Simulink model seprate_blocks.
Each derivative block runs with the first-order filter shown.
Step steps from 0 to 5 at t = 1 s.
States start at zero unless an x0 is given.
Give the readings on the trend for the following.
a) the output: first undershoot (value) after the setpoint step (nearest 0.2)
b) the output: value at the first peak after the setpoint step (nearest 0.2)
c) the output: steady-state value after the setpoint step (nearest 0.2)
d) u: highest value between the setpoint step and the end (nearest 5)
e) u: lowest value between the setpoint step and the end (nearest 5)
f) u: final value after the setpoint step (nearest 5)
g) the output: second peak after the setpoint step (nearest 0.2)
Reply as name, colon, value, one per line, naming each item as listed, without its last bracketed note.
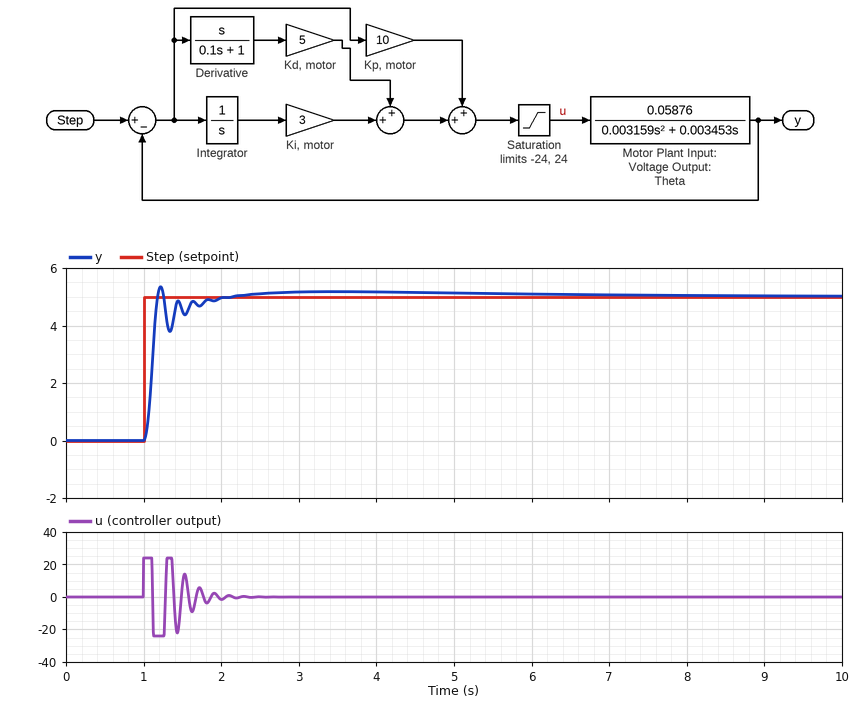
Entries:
the output: first undershoot (value) after the setpoint step: 3.8
the output: value at the first peak after the setpoint step: 5.4
the output: steady-state value after the setpoint step: 5.0
u: highest value between the setpoint step and the end: 25
u: lowest value between the setpoint step and the end: -25
u: final value after the setpoint step: 0
the output: second peak after the setpoint step: 4.8
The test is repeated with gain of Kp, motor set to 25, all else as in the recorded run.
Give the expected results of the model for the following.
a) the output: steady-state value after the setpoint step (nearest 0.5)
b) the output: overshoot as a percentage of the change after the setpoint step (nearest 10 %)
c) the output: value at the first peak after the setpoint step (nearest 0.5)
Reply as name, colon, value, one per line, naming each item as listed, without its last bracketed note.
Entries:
the output: steady-state value after the setpoint step: 5.0
the output: overshoot as a percentage of the change after the setpoint step: 20 %
the output: value at the first peak after the setpoint step: 6.0
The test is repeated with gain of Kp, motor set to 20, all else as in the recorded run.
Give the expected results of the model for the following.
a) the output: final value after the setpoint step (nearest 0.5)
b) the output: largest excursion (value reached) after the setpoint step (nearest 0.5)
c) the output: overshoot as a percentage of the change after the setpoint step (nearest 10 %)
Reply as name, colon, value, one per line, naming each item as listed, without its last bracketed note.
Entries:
the output: final value after the setpoint step: 5.0
the output: largest excursion (value reached) after the setpoint step: 6.0
the output: overshoot as a percentage of the change after the setpoint step: 20 %
